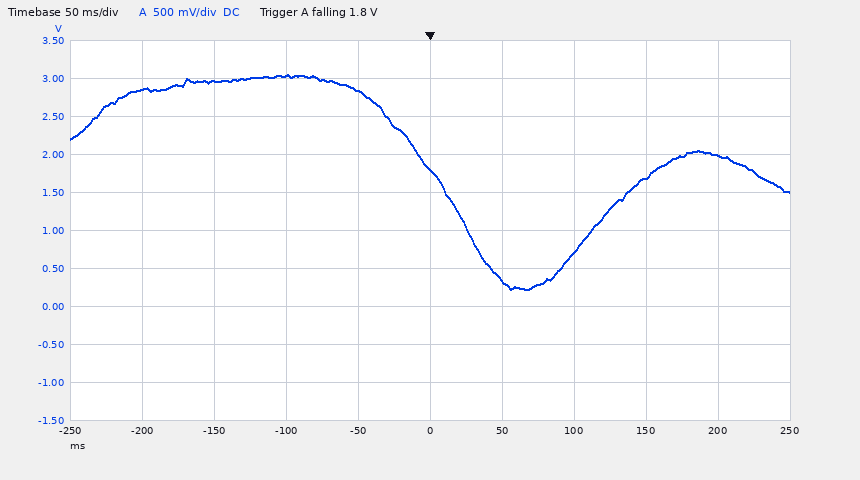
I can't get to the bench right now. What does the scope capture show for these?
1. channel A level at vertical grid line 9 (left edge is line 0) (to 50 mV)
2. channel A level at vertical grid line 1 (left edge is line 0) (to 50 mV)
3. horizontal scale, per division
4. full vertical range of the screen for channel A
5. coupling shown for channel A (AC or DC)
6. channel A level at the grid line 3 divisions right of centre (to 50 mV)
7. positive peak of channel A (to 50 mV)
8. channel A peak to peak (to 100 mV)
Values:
2.00 V
2.85 V
50 ms
5 V
DC
1.70 V
3.05 V
2.80 V
